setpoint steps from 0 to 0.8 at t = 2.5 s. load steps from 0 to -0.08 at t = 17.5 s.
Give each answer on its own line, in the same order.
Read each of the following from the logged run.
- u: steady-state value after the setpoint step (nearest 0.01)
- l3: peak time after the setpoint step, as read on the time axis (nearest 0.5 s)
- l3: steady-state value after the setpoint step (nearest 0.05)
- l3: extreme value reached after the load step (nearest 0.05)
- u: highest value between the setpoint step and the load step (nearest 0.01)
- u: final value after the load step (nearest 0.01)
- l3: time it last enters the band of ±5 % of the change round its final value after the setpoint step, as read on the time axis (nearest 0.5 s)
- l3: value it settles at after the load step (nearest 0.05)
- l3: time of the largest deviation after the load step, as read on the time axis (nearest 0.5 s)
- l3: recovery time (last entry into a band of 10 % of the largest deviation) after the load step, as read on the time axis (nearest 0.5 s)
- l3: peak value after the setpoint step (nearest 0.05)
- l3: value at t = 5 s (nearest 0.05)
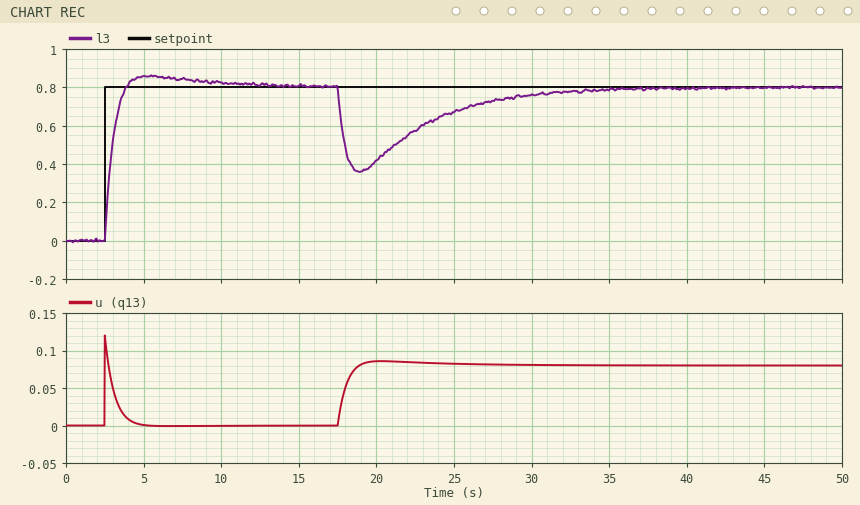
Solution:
0.00
5.5 s
0.80
0.35
0.12
0.08
7.5 s
0.80
19.0 s
29.5 s
0.85
0.85
